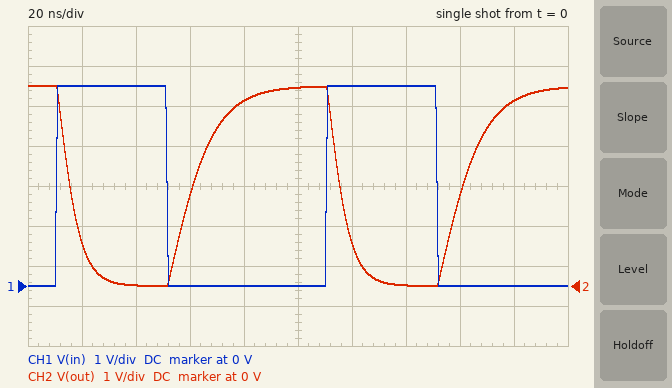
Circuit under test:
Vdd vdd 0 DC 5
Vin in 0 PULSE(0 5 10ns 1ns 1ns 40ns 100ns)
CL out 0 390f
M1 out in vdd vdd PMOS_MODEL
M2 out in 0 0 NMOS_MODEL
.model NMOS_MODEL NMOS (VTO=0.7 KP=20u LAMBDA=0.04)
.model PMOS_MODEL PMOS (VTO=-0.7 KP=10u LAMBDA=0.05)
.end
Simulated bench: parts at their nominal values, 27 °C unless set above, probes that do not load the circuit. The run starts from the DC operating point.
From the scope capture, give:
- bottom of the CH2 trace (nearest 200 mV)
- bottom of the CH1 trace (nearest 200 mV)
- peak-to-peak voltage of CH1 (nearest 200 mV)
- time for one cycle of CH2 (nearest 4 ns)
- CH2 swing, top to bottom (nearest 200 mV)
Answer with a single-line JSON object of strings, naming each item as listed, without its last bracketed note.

{"bottom of the CH2 trace": "0 V", "bottom of the CH1 trace": "0 V", "peak-to-peak voltage of CH1": "5.0 V", "time for one cycle of CH2": "100 ns", "CH2 swing, top to bottom": "5.0 V"}
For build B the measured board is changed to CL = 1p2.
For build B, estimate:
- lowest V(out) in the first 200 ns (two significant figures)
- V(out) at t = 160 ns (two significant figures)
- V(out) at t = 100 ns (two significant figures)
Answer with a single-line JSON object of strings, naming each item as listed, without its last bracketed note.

{"lowest V(out) in the first 200 ns": "350 mV", "V(out) at t = 160 ns": "1.1 V", "V(out) at t = 100 ns": "3.8 V"}
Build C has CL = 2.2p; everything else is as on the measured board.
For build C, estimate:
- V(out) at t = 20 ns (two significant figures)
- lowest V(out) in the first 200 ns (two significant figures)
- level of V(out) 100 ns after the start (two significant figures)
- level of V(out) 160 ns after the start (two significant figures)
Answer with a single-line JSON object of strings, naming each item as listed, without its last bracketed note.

{"V(out) at t = 20 ns": "4.1 V", "lowest V(out) in the first 200 ns": "1.0 V", "level of V(out) 100 ns after the start": "3.4 V", "level of V(out) 160 ns after the start": "1.4 V"}
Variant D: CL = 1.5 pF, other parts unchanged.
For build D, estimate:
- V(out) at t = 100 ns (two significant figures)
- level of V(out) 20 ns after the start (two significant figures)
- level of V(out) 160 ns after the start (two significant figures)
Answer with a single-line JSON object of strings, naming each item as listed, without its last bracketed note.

{"V(out) at t = 100 ns": "3.6 V", "level of V(out) 20 ns after the start": "3.7 V", "level of V(out) 160 ns after the start": "1.2 V"}
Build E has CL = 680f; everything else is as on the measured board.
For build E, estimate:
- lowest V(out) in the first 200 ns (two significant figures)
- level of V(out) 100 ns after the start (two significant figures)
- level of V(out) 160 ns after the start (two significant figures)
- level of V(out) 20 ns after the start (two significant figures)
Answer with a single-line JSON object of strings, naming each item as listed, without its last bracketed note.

{"lowest V(out) in the first 200 ns": "50 mV", "level of V(out) 100 ns after the start": "4.6 V", "level of V(out) 160 ns after the start": "1.4 V", "level of V(out) 20 ns after the start": "2.3 V"}
